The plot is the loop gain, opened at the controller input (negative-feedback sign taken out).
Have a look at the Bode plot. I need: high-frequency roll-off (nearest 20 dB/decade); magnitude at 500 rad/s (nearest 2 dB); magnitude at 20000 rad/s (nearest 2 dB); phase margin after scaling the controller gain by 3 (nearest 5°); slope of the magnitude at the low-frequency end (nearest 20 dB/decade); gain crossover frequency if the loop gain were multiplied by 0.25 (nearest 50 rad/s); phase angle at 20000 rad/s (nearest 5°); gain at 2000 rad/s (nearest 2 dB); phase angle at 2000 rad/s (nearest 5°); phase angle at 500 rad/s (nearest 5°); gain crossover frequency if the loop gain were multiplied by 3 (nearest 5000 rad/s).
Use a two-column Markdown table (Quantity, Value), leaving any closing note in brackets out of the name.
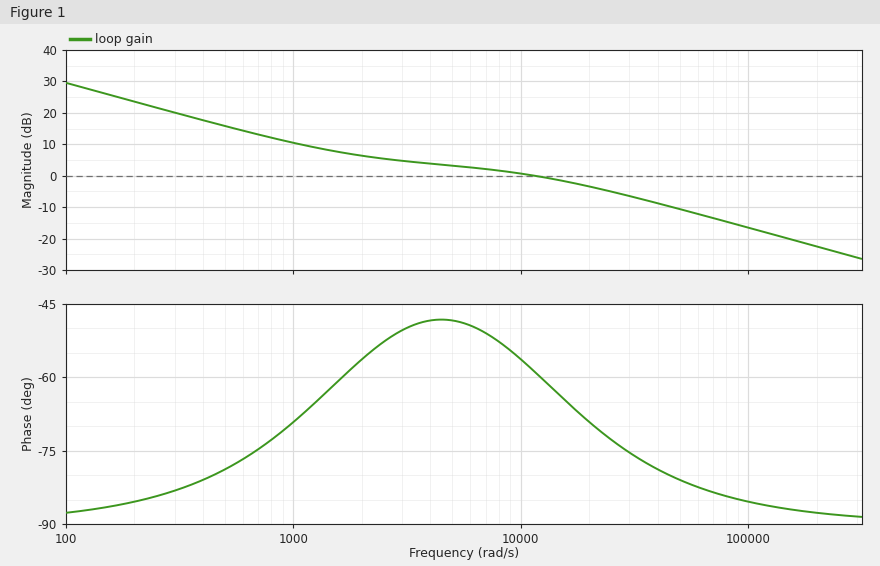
| Quantity | Value |
|---|---|
| high-frequency roll-off | -20 dB/decade |
| magnitude at 500 rad/s | 16 dB |
| magnitude at 20000 rad/s | -4 dB |
| phase margin after scaling the controller gain by 3 | 100° |
| slope of the magnitude at the low-frequency end | -20 dB/decade |
| gain crossover frequency if the loop gain were multiplied by 0.25 | 800 rad/s |
| phase angle at 20000 rad/s | -70° |
| gain at 2000 rad/s | 6 dB |
| phase angle at 2000 rad/s | -55° |
| phase angle at 500 rad/s | -80° |
| gain crossover frequency if the loop gain were multiplied by 3 | 45000 rad/s |
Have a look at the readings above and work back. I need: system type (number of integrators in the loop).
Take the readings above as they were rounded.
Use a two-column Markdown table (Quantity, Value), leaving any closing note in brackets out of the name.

| Quantity | Value |
|---|---|
| system type | 1 |
